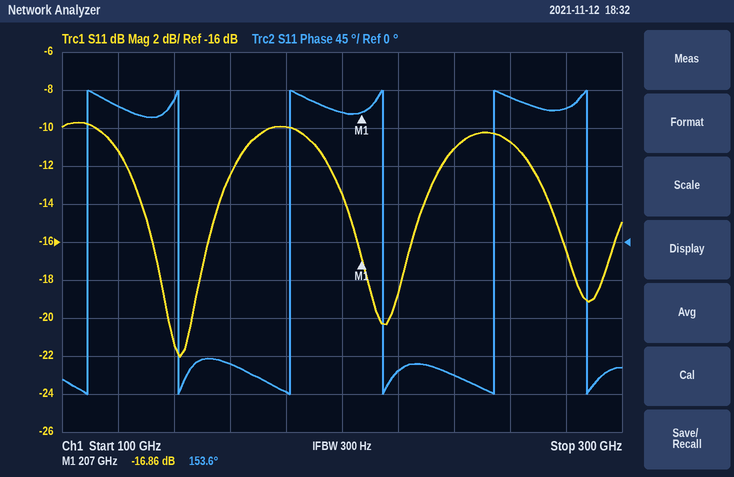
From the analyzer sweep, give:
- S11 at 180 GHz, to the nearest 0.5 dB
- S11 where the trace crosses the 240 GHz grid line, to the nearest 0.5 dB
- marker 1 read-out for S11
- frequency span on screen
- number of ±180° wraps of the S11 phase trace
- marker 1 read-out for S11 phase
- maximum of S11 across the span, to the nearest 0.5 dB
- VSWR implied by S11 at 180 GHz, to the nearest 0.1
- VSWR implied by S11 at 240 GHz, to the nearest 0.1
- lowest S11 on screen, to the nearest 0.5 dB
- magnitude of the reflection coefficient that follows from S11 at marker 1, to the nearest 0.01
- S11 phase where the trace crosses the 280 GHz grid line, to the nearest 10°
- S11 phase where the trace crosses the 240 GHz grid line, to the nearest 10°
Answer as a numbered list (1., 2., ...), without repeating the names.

1. -10.0 dB
2. -11.0 dB
3. -16.86 dB
4. 200 GHz
5. 6
6. 153.6°
7. -9.5 dB
8. 1.9
9. 1.8
10. -22.0 dB
11. 0.14
12. 160°
13. -160°
